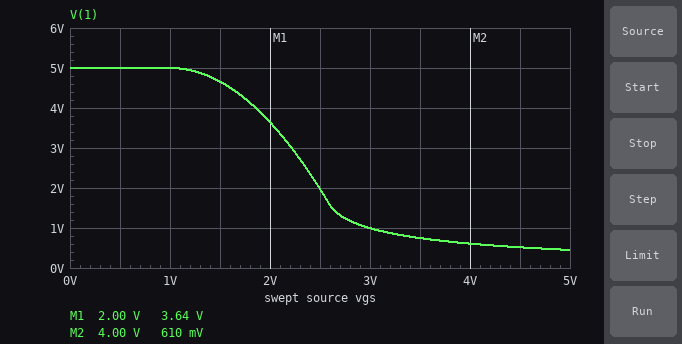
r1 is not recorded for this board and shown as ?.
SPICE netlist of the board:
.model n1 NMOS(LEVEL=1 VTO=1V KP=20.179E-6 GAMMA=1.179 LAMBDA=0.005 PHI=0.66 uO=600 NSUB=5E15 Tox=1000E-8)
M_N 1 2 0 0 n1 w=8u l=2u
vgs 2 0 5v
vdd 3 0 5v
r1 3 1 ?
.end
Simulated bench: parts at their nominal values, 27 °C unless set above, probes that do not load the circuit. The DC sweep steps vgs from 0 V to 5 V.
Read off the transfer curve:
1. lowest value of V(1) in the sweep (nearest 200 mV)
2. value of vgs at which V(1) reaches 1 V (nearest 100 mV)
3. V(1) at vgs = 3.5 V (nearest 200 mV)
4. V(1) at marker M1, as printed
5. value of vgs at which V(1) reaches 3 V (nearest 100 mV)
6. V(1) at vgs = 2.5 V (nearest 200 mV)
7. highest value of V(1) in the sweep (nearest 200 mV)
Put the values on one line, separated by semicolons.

400 mV; 3.0 V; 800 mV; 3.64 V; 2.2 V; 2.0 V; 5.0 V
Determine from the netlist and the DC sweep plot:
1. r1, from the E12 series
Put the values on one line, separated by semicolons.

33 kΩ
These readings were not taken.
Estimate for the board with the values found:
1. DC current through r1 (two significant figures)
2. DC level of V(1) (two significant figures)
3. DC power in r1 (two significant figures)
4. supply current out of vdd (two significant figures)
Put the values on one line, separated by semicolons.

140 µA; 450 mV; 630 µW; 140 µA
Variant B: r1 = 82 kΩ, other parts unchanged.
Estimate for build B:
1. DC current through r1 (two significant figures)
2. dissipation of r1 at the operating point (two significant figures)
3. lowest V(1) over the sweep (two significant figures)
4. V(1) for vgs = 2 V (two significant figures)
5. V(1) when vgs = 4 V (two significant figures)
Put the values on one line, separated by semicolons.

59 µA; 280 µW; 190 mV; 1.7 V; 250 mV
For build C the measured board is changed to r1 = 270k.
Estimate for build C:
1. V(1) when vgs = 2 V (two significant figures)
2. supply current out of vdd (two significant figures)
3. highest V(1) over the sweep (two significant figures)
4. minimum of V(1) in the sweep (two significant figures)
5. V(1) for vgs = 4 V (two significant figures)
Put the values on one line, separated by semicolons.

250 mV; 18 µA; 5.0 V; 57 mV; 76 mV
